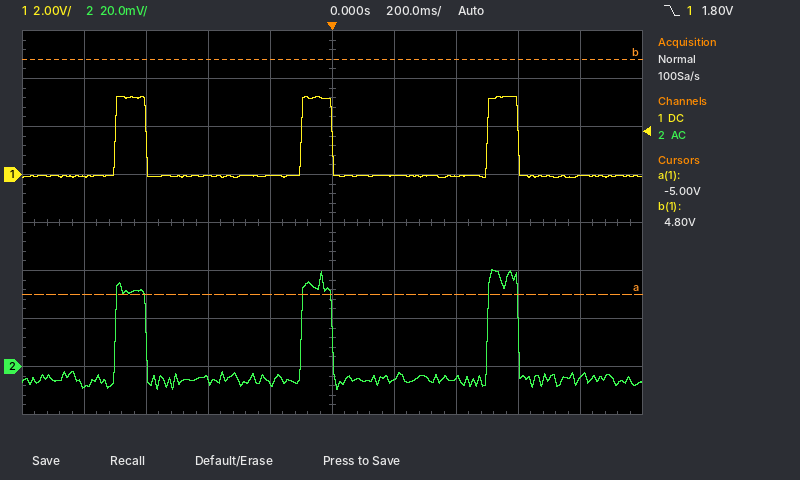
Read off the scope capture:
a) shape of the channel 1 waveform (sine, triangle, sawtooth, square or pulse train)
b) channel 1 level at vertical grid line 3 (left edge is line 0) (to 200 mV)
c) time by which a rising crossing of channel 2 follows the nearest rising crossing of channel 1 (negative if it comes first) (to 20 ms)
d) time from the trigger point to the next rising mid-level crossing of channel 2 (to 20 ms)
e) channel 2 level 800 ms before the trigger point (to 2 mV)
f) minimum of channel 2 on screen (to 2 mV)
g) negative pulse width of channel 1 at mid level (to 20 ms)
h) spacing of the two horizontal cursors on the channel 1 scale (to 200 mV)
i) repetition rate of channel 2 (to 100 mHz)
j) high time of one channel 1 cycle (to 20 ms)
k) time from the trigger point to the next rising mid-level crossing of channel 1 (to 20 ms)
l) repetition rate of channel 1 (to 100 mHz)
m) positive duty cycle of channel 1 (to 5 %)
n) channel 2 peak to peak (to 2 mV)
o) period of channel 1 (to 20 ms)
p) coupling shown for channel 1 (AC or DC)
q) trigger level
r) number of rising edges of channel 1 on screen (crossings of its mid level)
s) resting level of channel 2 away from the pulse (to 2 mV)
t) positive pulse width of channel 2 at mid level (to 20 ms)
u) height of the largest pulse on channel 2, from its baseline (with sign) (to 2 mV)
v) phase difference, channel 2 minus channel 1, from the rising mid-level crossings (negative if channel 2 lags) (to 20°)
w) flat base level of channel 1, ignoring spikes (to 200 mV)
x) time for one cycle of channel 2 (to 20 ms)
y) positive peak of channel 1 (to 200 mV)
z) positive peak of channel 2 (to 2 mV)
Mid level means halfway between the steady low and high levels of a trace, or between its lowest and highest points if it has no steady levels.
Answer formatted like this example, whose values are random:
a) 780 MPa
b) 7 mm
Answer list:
a) pulse train
b) 0.0 V
c) 0 ms
d) 500 ms
e) -8 mV
f) -10 mV
g) 500 ms
h) 9.8 V
i) 1.7 Hz
j) 100 ms
k) 500 ms
l) 1.7 Hz
m) 15 %
n) 50 mV
o) 600 ms
p) DC
q) 1.80 V
r) 3
s) -6 mV
t) 100 ms
u) +46 mV
v) 0°
w) 0.0 V
x) 600 ms
y) 3.2 V
z) 40 mV
